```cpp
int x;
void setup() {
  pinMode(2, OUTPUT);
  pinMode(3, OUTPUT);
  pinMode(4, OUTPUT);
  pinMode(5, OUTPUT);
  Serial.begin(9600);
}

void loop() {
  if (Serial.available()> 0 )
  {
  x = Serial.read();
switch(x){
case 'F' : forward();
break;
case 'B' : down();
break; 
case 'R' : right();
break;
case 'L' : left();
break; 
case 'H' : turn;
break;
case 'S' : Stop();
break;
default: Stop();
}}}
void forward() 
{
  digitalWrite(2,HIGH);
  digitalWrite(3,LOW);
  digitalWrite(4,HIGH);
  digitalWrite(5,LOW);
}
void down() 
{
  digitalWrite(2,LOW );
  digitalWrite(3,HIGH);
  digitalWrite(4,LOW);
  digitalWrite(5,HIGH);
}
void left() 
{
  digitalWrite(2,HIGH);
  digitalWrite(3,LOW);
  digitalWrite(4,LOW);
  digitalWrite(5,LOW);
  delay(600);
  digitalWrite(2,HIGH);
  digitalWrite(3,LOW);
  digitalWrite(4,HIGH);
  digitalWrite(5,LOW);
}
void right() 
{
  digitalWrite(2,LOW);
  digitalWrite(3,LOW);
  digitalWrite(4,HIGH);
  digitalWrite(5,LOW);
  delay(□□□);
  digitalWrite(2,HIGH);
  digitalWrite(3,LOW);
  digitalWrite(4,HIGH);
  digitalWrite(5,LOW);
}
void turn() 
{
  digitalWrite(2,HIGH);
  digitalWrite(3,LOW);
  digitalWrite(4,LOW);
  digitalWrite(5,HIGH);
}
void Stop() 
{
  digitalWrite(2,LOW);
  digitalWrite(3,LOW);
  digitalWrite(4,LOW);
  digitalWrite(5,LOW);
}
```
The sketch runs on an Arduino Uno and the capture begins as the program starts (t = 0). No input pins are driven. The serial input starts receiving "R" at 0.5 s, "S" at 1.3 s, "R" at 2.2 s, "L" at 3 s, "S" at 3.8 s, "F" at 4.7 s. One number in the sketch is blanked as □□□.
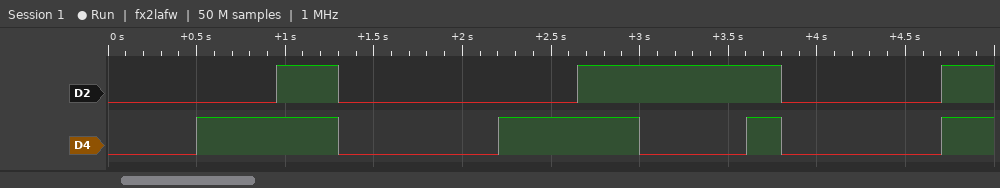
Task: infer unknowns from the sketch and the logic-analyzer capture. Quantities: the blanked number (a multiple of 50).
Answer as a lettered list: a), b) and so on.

a) 450
